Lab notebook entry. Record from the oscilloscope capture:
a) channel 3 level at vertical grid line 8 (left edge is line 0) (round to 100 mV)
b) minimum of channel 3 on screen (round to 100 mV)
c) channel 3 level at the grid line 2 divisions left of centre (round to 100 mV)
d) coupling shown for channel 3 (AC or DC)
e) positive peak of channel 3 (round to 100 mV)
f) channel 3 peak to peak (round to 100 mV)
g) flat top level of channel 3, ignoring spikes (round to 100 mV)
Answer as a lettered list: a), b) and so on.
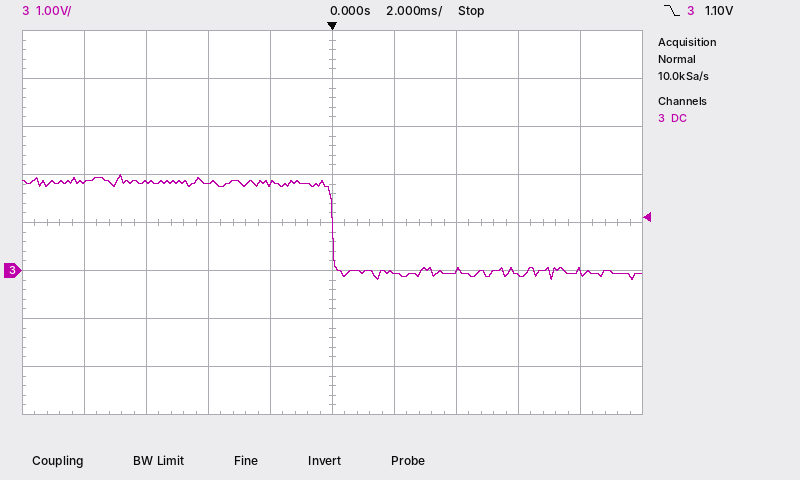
a) -100 mV
b) -200 mV
c) 1.8 V
d) DC
e) 2.0 V
f) 2.2 V
g) 1.8 V
